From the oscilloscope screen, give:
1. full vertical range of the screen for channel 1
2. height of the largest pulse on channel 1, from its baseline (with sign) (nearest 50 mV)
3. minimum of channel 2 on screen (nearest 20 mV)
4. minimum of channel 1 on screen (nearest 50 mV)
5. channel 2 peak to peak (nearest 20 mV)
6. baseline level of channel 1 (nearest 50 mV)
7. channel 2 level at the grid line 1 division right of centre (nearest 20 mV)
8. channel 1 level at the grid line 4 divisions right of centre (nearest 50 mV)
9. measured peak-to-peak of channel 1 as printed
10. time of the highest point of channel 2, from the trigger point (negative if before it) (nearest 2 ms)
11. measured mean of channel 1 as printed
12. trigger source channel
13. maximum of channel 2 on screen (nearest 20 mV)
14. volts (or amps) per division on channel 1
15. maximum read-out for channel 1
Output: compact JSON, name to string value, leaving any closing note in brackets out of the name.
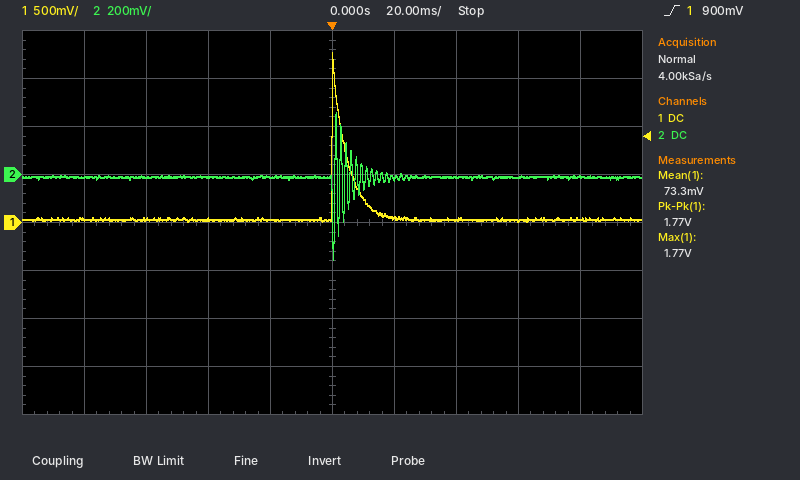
{"full vertical range of the screen for channel 1": "4 V", "height of the largest pulse on channel 1, from its baseline (with sign)": "+1.75 V", "minimum of channel 2 on screen": "-360 mV", "minimum of channel 1 on screen": "0 mV", "channel 2 peak to peak": "620 mV", "baseline level of channel 1": "50 mV", "channel 2 level at the grid line 1 division right of centre": "-20 mV", "channel 1 level at the grid line 4 divisions right of centre": "50 mV", "measured peak-to-peak of channel 1 as printed": "1.77 V", "time of the highest point of channel 2, from the trigger point (negative if before it)": "+2 ms", "measured mean of channel 1 as printed": "73.3 mV", "trigger source channel": "channel 1", "maximum of channel 2 on screen": "260 mV", "volts (or amps) per division on channel 1": "500 mV", "maximum read-out for channel 1": "1.77 V"}
